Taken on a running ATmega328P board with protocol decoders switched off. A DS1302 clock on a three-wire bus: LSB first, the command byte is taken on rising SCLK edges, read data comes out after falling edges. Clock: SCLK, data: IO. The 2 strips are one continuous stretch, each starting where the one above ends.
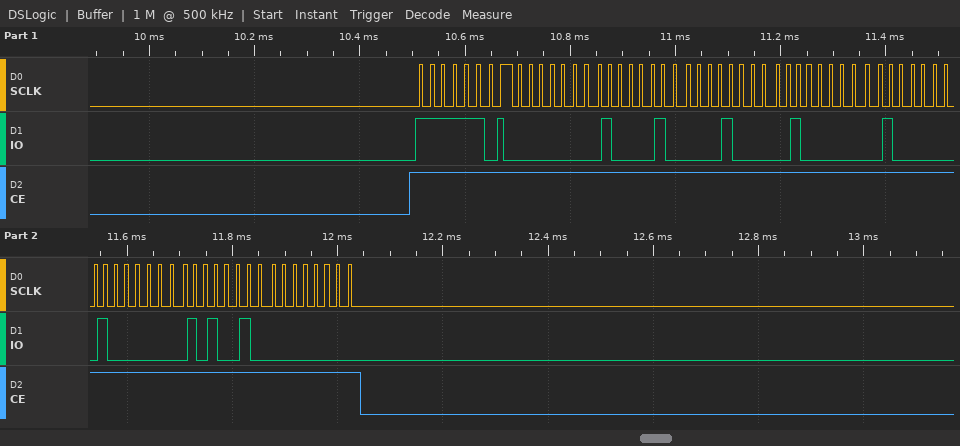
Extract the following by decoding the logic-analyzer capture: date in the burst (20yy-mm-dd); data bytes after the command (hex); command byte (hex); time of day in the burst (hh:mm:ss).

2025-02-02
00 21 08 02 02 01 25 00
0xBF
08:21:00
